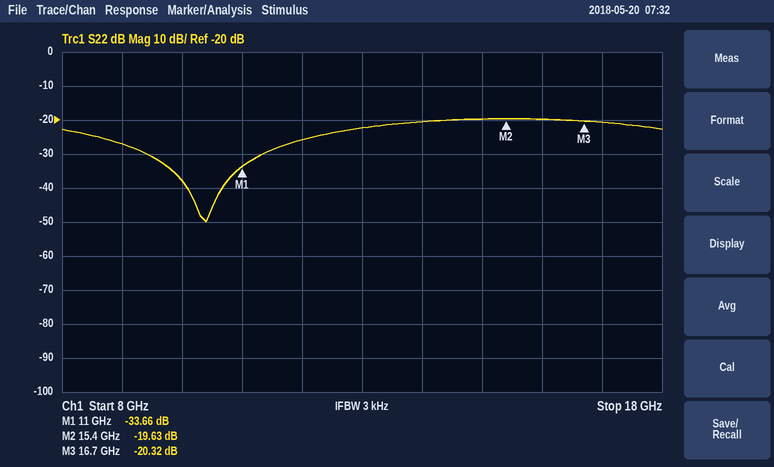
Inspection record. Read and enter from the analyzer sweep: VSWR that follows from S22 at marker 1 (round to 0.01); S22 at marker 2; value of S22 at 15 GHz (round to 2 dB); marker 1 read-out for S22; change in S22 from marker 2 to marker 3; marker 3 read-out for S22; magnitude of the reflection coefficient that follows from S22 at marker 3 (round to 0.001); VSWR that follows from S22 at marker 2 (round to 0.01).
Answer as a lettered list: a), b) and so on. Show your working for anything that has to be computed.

a) (1 + 0.0207)/(1 − 0.0207) ≈ 1.04
b) -19.63 dB
c) -20 dB
d) -33.66 dB
e) -20.32 − (-19.63) = -0.69 dB
f) -20.32 dB
g) 10^(-20.32/20) ≈ 0.096
h) (1 + 0.1044)/(1 − 0.1044) ≈ 1.23
